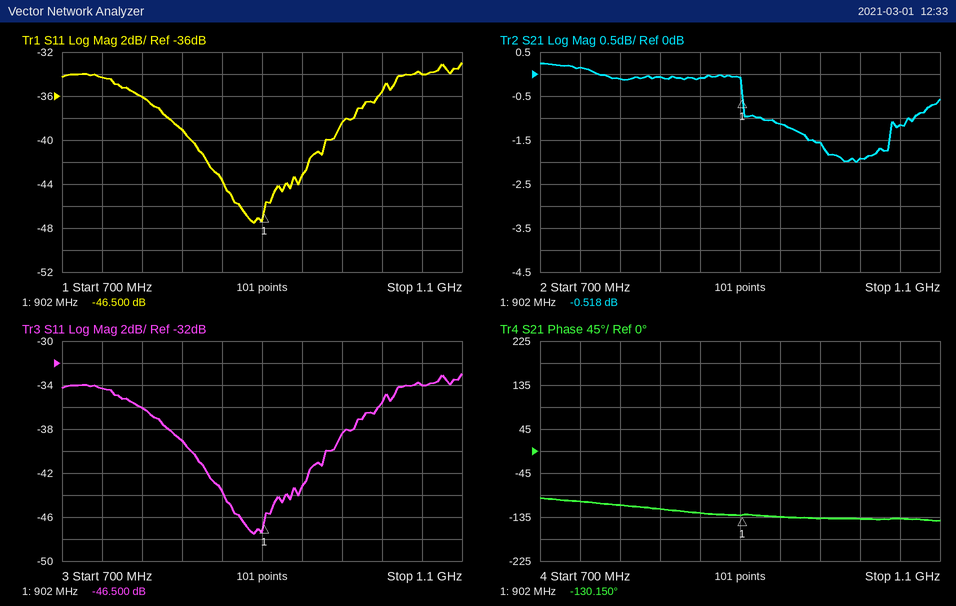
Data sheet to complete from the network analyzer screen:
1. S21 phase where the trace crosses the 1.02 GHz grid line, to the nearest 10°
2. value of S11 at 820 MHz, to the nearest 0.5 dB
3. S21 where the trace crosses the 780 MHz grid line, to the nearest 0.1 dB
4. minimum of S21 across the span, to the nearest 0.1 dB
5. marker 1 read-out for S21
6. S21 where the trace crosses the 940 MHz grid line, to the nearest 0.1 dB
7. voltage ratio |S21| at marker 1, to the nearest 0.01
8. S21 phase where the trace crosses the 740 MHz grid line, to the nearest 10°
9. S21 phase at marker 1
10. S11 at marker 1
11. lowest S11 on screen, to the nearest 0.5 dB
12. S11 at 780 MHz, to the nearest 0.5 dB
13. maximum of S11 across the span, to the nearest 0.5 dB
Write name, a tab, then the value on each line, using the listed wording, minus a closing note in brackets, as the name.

S21 phase where the trace crosses the 1.02 GHz grid line, to the nearest 10°	-140°
value of S11 at 820 MHz, to the nearest 0.5 dB	-39.0 dB
S21 where the trace crosses the 780 MHz grid line, to the nearest 0.1 dB	-0.1 dB
minimum of S21 across the span, to the nearest 0.1 dB	-2.0 dB
marker 1 read-out for S21	-0.518 dB
S21 where the trace crosses the 940 MHz grid line, to the nearest 0.1 dB	-1.1 dB
voltage ratio |S21| at marker 1, to the nearest 0.01	0.94
S21 phase where the trace crosses the 740 MHz grid line, to the nearest 10°	-100°
S21 phase at marker 1	-130.150°
S11 at marker 1	-46.500 dB
lowest S11 on screen, to the nearest 0.5 dB	-47.5 dB
S11 at 780 MHz, to the nearest 0.5 dB	-36.0 dB
maximum of S11 across the span, to the nearest 0.5 dB	-33.0 dB
